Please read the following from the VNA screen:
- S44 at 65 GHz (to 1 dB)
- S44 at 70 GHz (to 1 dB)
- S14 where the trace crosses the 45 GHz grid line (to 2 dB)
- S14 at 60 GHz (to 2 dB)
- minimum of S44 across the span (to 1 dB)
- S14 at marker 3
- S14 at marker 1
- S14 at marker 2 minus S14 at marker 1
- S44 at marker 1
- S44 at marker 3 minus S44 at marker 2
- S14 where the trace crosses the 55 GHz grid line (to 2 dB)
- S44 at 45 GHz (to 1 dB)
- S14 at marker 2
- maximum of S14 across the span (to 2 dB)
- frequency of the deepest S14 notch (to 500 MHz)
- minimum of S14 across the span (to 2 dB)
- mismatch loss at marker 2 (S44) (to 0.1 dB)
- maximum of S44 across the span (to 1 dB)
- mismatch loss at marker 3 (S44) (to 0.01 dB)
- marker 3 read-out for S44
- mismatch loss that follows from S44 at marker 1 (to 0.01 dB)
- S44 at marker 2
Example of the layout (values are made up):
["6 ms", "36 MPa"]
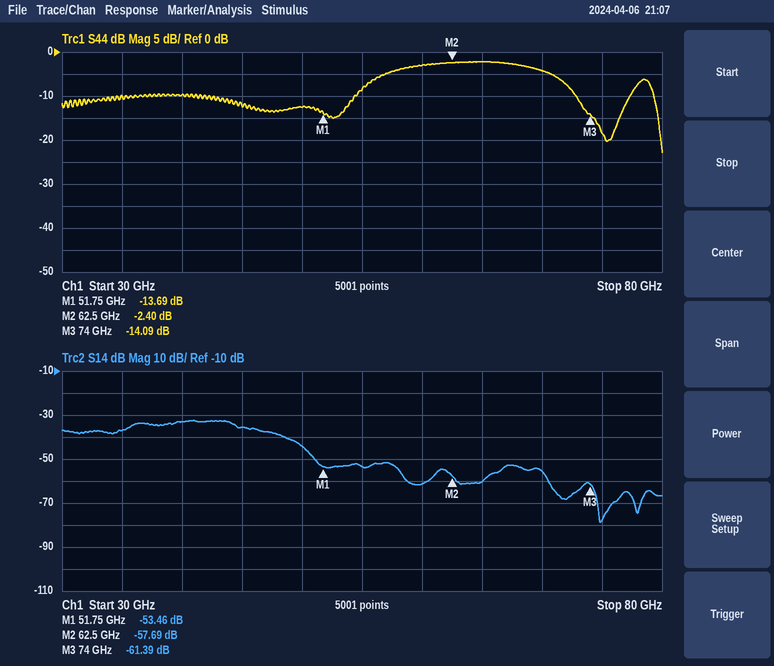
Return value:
["-2 dB", "-4 dB", "-36 dB", "-62 dB", "-23 dB", "-61.39 dB", "-53.46 dB", "-4.23 dB", "-13.69 dB", "-11.69 dB", "-54 dB", "-12 dB", "-57.69 dB", "-32 dB", "75.0 GHz", "-78 dB", "3.7 dB", "-2 dB", "0.17 dB", "-14.09 dB", "0.19 dB", "-2.40 dB"]
